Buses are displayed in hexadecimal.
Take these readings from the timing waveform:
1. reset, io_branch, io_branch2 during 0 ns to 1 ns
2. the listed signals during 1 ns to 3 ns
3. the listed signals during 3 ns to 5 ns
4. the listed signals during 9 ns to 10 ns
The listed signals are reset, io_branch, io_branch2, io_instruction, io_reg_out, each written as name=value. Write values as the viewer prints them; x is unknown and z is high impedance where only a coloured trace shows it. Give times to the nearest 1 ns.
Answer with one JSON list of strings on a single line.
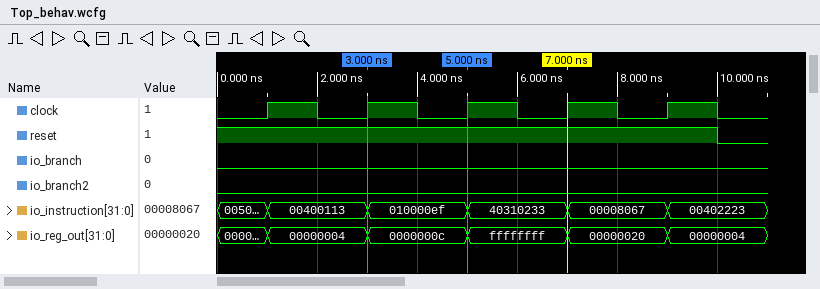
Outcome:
["reset=1, io_branch=0, io_branch2=0", "reset=1, io_branch=0, io_branch2=0, io_instruction=00400113, io_reg_out=00000004", "reset=1, io_branch=0, io_branch2=0, io_instruction=010000ef, io_reg_out=0000000c", "reset=1, io_branch=0, io_branch2=0, io_instruction=00402223, io_reg_out=00000004"]
